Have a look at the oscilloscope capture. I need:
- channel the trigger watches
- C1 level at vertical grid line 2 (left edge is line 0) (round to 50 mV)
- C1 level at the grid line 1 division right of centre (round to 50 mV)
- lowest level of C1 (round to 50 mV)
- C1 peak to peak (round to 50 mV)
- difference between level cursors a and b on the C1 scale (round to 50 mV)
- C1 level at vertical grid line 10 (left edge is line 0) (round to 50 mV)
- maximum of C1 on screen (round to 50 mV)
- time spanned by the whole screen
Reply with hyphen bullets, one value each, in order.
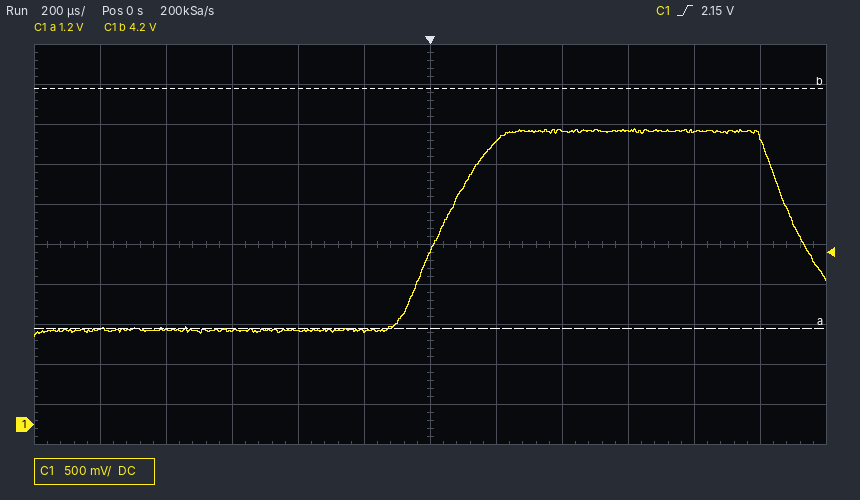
- C1
- 1.20 V
- 3.55 V
- 1.10 V
- 2.60 V
- 3.00 V
- 3.65 V
- 3.70 V
- 2.4 ms
